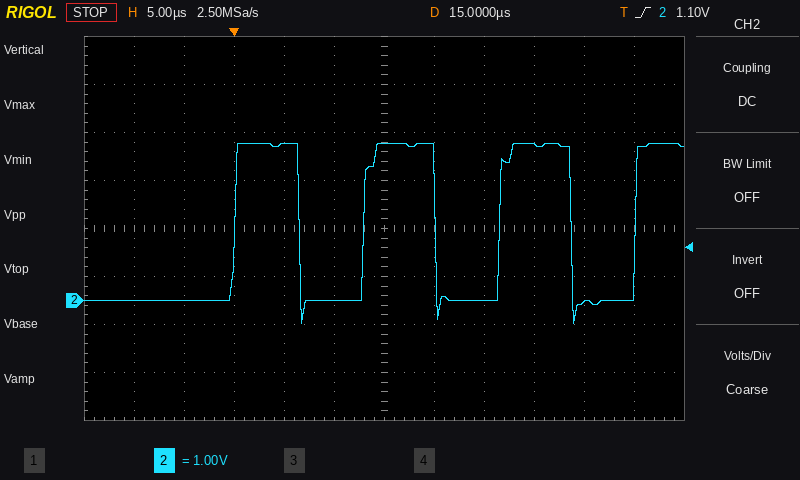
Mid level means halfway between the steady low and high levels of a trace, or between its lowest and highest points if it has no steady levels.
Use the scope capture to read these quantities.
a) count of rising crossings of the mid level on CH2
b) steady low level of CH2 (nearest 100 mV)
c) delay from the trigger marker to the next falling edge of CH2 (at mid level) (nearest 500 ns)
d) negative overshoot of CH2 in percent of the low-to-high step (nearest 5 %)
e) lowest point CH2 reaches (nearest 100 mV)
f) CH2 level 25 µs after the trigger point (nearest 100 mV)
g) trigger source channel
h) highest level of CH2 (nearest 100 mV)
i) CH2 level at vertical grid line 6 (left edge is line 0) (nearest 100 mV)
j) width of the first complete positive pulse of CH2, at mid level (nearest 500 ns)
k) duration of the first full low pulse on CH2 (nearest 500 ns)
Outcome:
4
0.0 V
6.5 µs
15 %
-500 mV
0.0 V
CH2
3.3 V
3.3 V
6.5 µs
6.5 µs
